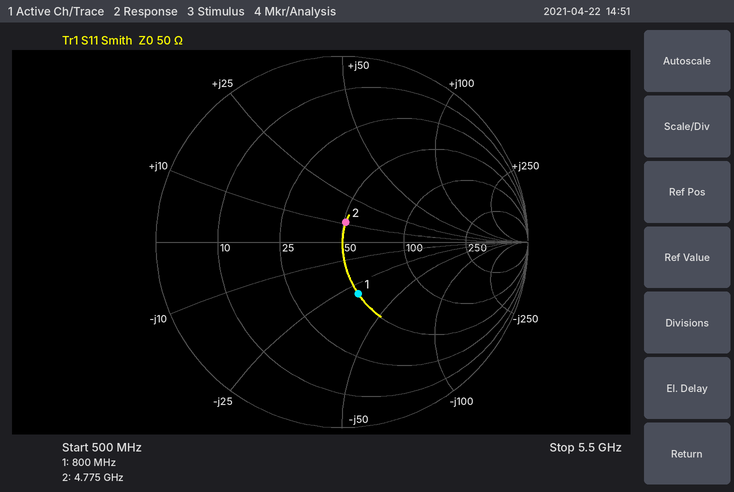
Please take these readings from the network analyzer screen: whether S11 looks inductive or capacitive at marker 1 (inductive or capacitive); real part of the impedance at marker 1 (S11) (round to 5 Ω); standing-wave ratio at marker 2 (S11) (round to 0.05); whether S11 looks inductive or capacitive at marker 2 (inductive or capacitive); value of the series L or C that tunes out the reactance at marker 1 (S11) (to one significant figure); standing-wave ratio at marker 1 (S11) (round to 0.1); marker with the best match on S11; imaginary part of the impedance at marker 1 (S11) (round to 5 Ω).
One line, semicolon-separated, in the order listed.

capacitive; 50 Ω; 1.25; inductive; 6 nH; 1.8; marker 2; -30 Ω
